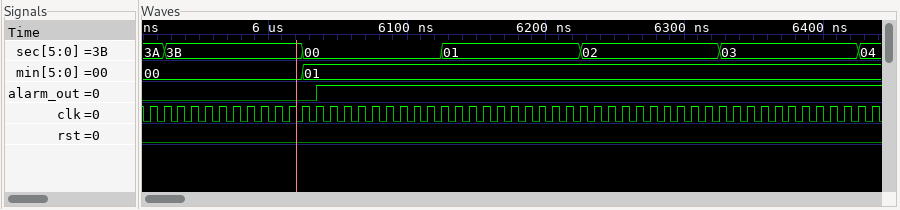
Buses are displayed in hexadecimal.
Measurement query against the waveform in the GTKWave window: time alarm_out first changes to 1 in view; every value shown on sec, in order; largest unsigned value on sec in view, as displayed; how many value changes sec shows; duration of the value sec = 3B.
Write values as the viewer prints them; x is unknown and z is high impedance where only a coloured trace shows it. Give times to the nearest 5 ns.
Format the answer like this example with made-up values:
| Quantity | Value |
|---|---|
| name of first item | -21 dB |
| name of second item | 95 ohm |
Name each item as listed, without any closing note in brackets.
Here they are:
| Quantity | Value |
|---|---|
| time alarm_out first changes to 1 in view | 6035 ns |
| every value shown on sec, in order | 3A, 3B, 00, 01, 02, 03, 04 |
| largest unsigned value on sec in view, as displayed | 3B |
| how many value changes sec shows | 6 |
| duration of the value sec = 3B | 100 ns |
